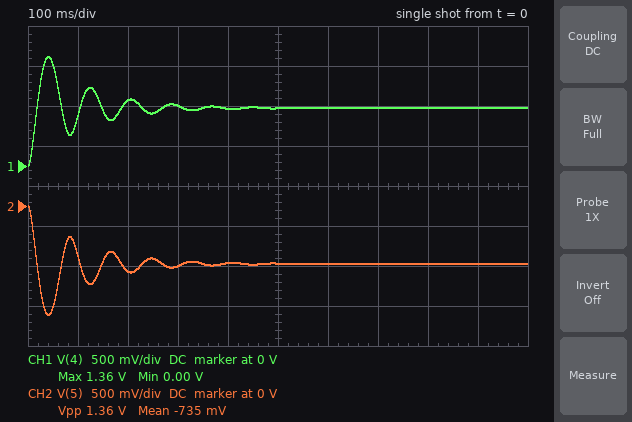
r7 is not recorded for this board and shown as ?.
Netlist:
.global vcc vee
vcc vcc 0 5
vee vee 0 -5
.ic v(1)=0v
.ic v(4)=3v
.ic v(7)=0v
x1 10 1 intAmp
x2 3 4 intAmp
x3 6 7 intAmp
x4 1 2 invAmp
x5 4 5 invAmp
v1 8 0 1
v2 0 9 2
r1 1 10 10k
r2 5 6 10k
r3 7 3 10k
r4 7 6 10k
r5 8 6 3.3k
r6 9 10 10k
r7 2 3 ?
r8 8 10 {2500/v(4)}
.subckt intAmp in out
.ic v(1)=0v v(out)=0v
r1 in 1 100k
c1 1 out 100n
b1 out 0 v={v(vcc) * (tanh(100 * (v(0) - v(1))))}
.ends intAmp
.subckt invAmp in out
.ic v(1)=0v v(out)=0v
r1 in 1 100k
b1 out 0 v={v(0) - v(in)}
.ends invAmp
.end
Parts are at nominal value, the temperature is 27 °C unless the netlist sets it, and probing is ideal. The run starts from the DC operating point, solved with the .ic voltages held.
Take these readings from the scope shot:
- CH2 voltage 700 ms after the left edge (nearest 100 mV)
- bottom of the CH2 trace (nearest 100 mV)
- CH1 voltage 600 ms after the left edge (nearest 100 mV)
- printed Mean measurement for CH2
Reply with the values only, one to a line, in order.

-700 mV
-1.4 V
700 mV
-735 mV
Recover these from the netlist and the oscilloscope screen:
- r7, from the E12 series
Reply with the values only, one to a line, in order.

3.9 kΩ
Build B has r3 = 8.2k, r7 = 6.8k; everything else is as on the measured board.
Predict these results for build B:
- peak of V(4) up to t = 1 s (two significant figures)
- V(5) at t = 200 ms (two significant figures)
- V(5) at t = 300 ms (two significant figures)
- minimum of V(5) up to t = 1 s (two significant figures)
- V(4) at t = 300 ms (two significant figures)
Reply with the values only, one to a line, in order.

1.8 V
-750 mV
-860 mV
-1.8 V
860 mV
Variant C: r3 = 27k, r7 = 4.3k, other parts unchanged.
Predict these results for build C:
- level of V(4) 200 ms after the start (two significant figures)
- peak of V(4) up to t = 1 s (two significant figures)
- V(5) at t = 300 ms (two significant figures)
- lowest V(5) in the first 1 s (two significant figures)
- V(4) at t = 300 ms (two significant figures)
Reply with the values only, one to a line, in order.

610 mV
1.1 V
-580 mV
-1.1 V
580 mV
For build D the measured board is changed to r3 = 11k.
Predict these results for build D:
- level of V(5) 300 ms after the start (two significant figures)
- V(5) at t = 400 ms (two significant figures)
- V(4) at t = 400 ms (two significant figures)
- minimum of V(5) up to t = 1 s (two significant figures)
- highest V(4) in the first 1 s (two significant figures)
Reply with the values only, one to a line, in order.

-720 mV
-690 mV
690 mV
-1.3 V
1.3 V
